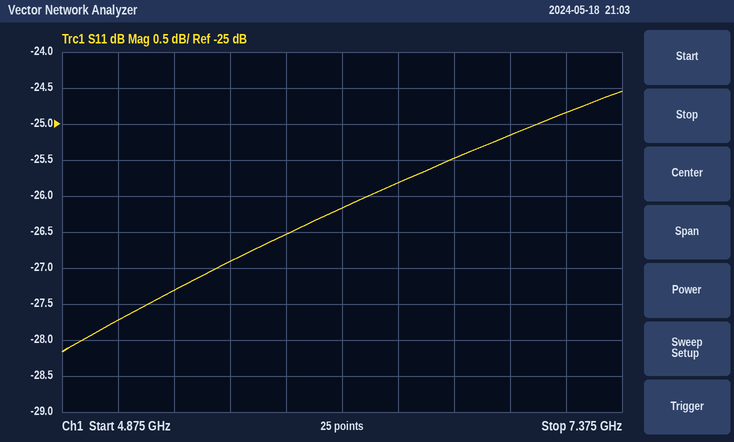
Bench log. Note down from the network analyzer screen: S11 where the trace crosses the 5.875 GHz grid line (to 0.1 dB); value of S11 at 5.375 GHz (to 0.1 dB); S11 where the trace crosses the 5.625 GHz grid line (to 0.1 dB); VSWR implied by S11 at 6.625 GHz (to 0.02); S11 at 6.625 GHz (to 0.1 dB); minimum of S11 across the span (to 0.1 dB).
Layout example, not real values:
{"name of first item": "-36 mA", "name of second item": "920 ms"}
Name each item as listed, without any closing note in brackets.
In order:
{"S11 where the trace crosses the 5.875 GHz grid line": "-26.5 dB", "value of S11 at 5.375 GHz": "-27.3 dB", "S11 where the trace crosses the 5.625 GHz grid line": "-26.9 dB", "VSWR implied by S11 at 6.625 GHz": "1.12", "S11 at 6.625 GHz": "-25.5 dB", "minimum of S11 across the span": "-28.2 dB"}
